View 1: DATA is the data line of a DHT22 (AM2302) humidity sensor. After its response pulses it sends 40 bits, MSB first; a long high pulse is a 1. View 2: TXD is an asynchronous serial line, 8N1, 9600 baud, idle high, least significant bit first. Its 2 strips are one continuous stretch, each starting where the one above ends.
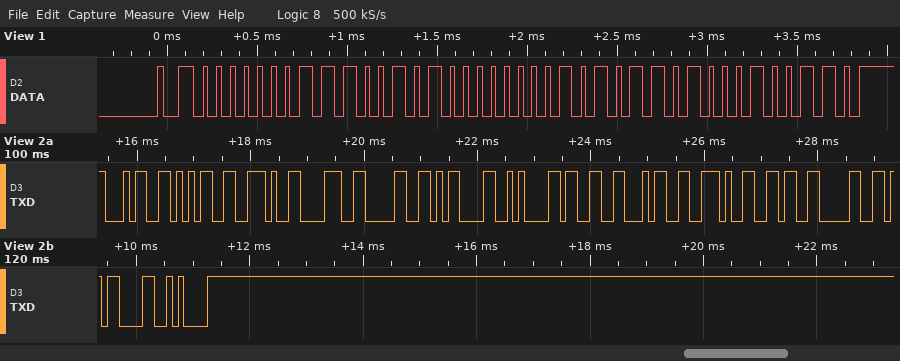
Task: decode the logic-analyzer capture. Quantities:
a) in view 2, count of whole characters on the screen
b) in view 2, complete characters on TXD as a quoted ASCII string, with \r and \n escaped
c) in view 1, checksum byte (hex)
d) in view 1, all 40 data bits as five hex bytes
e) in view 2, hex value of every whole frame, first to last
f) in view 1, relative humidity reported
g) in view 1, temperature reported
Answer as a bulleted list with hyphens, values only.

- 14
- "45.80\r\n34.60\r\n"
- 0x26
- 01 CA 01 5A 26
- 34 35 2E 38 30 0D 0A 33 34 2E 36 30 0D 0A
- 45.8 %
- 34.6 °C
